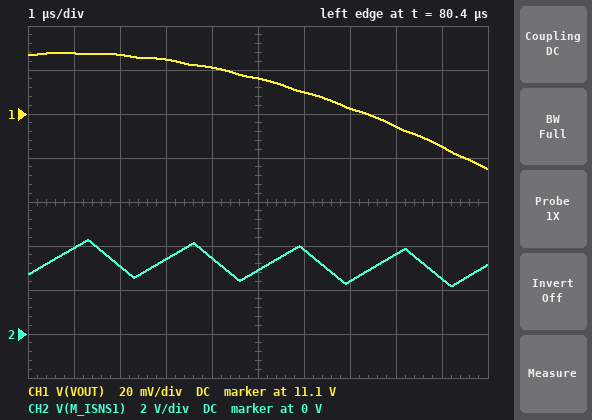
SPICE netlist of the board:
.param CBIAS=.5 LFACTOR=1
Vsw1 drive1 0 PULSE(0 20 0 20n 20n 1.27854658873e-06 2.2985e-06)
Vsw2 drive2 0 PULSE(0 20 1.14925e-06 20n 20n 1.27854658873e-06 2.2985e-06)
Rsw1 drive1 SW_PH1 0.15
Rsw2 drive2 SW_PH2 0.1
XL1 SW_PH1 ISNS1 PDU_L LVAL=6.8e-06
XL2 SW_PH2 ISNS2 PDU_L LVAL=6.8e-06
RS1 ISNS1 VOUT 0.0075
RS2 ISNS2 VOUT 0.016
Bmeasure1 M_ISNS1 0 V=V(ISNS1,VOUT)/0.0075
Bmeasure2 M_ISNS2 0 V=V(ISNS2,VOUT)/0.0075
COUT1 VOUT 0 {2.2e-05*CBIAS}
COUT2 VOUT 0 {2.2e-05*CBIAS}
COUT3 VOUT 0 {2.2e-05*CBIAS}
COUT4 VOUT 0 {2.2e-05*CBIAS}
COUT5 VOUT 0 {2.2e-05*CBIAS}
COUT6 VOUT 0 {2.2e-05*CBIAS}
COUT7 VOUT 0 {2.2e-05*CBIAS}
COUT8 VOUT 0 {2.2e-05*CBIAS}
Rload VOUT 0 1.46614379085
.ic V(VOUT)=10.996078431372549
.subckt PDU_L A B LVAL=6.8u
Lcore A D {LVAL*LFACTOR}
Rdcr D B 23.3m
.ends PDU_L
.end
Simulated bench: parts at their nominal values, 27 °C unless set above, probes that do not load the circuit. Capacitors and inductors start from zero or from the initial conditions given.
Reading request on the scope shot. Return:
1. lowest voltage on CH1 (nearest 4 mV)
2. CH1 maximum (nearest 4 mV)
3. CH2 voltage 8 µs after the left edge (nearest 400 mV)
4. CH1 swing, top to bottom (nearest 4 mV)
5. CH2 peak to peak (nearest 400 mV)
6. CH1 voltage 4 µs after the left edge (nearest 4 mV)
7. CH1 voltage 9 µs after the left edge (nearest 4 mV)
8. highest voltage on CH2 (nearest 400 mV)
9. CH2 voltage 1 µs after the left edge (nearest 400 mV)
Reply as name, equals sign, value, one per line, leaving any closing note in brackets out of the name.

lowest voltage on CH1 = 11.076 V
CH1 maximum = 11.128 V
CH2 voltage 8 µs after the left edge = 3.6 V
CH1 swing, top to bottom = 52 mV
CH2 peak to peak = 2.0 V
CH1 voltage 4 µs after the left edge = 11.120 V
CH1 voltage 9 µs after the left edge = 11.084 V
highest voltage on CH2 = 4.4 V
CH2 voltage 1 µs after the left edge = 4.0 V
